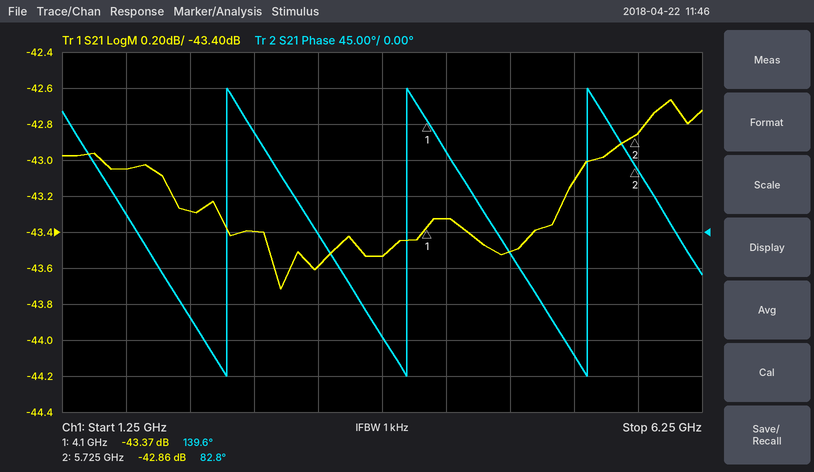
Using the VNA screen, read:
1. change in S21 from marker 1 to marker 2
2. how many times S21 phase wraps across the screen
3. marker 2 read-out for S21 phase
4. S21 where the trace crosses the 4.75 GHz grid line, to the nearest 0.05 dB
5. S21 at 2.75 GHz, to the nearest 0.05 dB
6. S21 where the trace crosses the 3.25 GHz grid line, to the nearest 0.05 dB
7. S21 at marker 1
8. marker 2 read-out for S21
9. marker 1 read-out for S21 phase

0.51 dB
3
82.8°
-43.50 dB
-43.40 dB
-43.60 dB
-43.37 dB
-42.86 dB
139.6°
